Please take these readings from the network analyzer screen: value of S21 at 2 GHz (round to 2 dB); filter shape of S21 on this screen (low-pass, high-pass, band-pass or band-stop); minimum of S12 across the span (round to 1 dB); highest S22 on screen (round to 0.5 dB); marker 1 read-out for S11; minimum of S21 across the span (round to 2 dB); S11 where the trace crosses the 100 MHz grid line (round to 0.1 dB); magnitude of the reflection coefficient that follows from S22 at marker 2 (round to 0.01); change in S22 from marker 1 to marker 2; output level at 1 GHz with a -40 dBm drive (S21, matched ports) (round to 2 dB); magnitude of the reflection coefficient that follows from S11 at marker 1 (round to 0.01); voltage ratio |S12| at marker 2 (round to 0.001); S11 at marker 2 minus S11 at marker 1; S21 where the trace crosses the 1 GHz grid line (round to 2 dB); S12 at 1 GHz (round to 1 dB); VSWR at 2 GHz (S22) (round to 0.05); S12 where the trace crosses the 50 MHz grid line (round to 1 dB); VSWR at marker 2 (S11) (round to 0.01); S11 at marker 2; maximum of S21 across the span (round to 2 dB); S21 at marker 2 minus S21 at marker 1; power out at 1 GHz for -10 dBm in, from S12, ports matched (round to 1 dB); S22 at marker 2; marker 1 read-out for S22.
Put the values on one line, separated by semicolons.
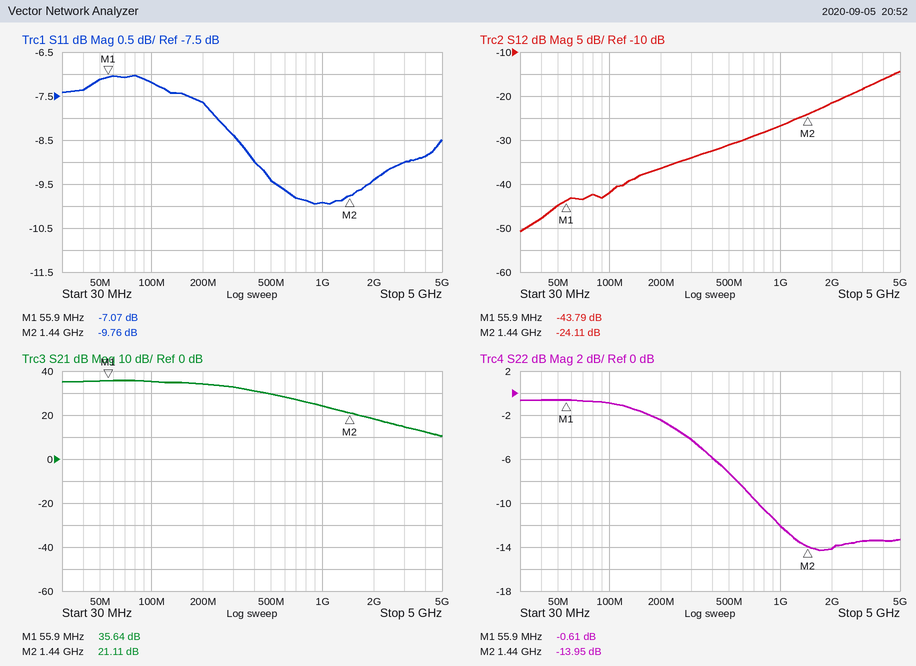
18 dB; low-pass; -51 dB; -0.5 dB; -7.07 dB; 10 dB; -7.2 dB; 0.20; -13.34 dB; -16 dBm; 0.44; 0.062; -2.69 dB; 24 dB; -27 dB; 1.50; -45 dB; 1.96; -9.76 dB; 36 dB; -14.53 dB; -37 dBm; -13.95 dB; -0.61 dB
